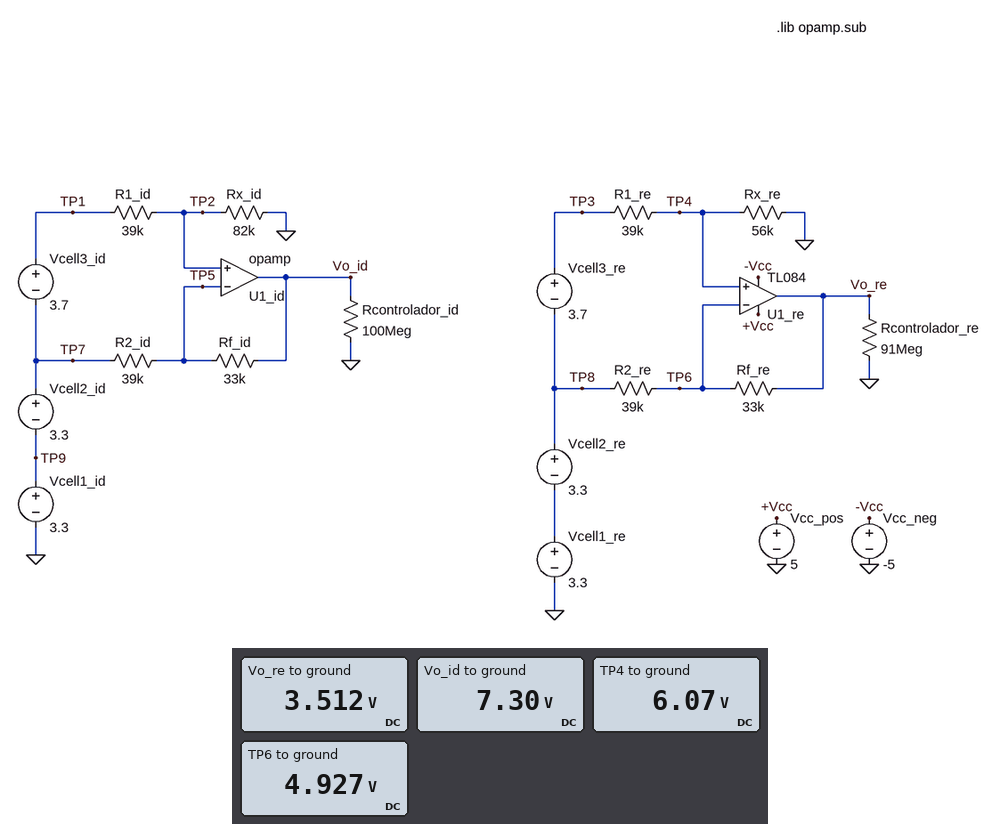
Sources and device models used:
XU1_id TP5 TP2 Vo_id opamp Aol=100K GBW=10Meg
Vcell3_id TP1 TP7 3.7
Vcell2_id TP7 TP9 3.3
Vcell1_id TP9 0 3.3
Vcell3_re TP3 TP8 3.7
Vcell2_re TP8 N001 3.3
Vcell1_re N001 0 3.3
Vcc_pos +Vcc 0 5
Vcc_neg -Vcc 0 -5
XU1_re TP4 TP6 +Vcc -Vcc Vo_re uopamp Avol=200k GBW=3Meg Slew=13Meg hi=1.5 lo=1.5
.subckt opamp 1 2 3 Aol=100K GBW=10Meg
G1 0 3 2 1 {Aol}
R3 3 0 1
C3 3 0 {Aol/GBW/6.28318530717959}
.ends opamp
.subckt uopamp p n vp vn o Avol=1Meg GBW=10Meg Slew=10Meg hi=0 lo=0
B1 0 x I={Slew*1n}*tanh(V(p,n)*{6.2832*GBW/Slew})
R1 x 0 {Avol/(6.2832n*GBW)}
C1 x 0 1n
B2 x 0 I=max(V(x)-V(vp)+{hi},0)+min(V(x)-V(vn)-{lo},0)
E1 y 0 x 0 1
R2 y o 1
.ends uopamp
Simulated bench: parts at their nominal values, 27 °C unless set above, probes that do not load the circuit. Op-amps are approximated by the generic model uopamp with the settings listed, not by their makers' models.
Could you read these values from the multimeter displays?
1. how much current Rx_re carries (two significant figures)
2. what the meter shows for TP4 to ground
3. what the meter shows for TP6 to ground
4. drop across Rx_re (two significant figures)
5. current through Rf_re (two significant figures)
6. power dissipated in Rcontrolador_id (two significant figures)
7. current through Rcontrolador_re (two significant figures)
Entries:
110 µA
6.07 V
4.927 V
6.1 V
43 µA
530 nW
39 nA
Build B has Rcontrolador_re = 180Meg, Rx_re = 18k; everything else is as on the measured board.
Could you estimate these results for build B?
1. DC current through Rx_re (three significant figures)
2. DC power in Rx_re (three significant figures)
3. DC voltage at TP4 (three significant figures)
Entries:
181 µA
588 µW
3.25 V
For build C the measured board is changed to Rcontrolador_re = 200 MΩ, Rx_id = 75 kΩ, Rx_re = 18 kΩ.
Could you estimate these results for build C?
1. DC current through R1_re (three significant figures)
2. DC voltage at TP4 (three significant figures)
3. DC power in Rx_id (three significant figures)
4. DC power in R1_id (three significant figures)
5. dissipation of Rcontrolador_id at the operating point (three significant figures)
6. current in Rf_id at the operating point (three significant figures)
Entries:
181 µA
3.25 V
612 µW
318 µW
480 nW
4.52 µA
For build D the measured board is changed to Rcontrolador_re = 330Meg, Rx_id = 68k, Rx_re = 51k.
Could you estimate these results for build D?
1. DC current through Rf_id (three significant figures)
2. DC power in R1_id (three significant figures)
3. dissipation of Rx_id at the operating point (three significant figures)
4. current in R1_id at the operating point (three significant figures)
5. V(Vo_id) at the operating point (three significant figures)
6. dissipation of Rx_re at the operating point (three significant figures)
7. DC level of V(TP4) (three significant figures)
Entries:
1.39 µA
361 µW
630 µW
96.3 µA
6.50 V
668 µW
5.84 V
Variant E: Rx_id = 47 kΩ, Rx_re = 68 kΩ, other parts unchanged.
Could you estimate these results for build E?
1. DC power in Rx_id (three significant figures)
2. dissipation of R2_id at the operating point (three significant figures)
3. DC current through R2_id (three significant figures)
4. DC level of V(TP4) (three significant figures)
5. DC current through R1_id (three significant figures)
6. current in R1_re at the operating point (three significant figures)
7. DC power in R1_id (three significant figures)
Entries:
674 µW
24.2 µW
24.9 µA
6.55 V
120 µA
96.3 µA
559 µW
